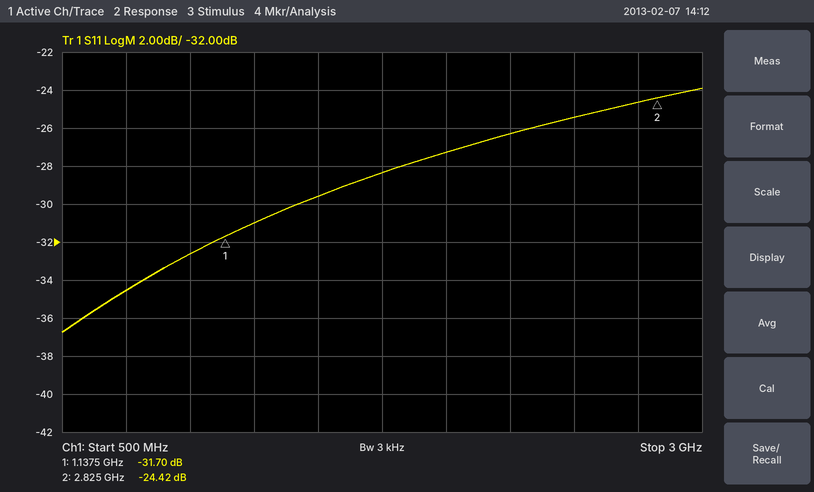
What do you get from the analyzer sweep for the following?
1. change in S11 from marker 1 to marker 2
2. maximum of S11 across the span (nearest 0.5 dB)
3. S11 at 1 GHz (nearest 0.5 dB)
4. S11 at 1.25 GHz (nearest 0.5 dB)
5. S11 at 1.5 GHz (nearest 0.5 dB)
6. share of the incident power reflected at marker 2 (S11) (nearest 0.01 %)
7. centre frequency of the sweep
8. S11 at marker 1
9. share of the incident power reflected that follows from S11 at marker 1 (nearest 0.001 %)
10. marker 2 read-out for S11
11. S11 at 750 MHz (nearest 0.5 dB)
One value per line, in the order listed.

7.28 dB
-24.0 dB
-32.5 dB
-31.0 dB
-29.5 dB
0.36 %
1.75 GHz
-31.70 dB
0.068 %
-24.42 dB
-34.5 dB
